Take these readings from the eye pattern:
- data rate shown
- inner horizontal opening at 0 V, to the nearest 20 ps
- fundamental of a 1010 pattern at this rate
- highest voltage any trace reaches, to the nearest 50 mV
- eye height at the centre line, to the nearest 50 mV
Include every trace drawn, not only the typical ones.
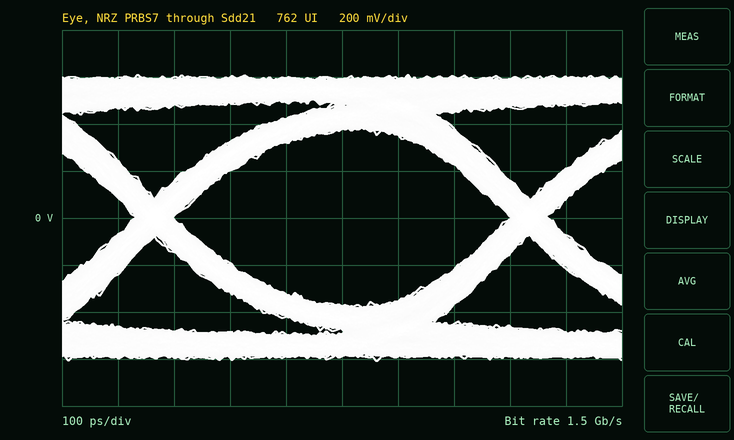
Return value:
1.5 Gb/s
600 ps
750 MHz
600 mV
750 mV
